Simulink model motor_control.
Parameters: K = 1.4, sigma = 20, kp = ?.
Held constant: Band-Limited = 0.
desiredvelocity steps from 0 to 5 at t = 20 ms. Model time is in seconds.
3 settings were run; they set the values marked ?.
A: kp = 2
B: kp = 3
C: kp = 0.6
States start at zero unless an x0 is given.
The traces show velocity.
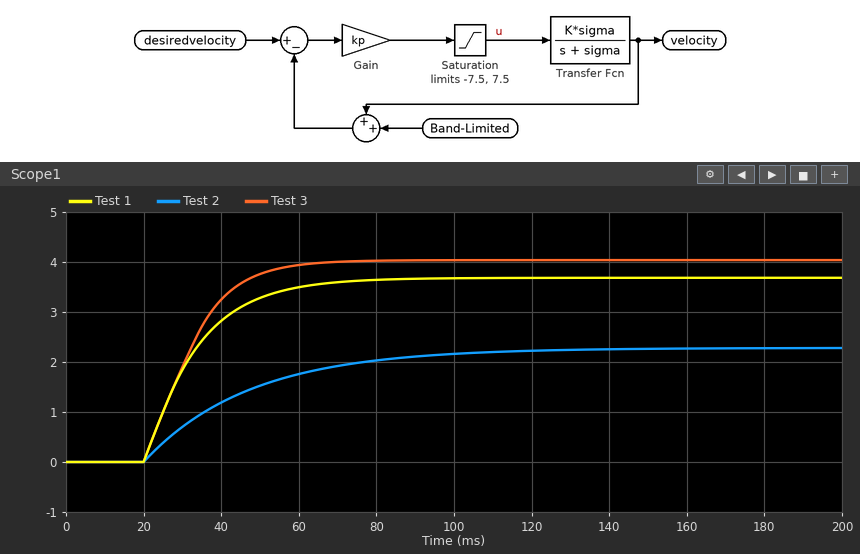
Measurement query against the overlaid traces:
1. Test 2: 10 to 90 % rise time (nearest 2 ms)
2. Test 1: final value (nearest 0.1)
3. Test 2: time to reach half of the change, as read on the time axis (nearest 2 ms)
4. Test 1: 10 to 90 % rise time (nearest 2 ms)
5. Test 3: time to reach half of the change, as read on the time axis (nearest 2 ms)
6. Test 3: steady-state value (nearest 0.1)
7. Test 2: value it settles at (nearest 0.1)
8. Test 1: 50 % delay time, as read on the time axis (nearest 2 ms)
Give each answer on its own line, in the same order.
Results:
60 ms
3.7
38 ms
30 ms
30 ms
4.0
2.3
30 ms
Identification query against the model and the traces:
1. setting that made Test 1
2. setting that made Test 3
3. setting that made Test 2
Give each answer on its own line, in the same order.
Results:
A
B
C
